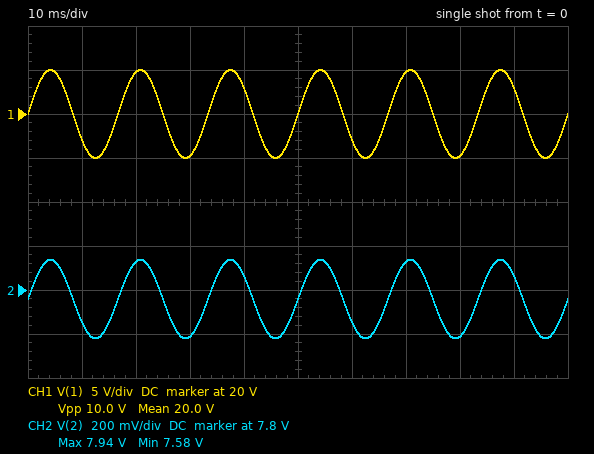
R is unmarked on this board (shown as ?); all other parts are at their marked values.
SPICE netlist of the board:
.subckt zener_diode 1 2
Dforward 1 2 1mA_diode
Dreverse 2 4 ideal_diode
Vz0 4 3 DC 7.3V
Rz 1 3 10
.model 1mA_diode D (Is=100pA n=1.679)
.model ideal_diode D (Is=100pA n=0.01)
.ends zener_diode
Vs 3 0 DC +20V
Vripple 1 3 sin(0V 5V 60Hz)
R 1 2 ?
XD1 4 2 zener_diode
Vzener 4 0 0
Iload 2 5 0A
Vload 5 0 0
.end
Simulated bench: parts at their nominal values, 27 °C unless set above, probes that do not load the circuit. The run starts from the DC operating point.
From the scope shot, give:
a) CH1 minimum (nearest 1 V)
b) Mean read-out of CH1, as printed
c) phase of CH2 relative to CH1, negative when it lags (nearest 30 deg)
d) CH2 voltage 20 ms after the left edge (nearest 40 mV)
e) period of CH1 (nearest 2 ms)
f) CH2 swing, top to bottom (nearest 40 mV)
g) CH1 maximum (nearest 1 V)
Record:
15 V
20.0 V
0 deg
7.92 V
16 ms
360 mV
25 V
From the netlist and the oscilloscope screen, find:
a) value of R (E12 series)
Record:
270 Ω
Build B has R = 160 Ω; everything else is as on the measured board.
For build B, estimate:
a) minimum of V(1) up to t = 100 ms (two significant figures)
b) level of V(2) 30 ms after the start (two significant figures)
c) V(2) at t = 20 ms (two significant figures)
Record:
15 V
7.8 V
8.3 V
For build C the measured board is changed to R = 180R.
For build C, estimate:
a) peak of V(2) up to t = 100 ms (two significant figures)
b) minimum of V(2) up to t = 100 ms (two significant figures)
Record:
8.2 V
7.7 V
